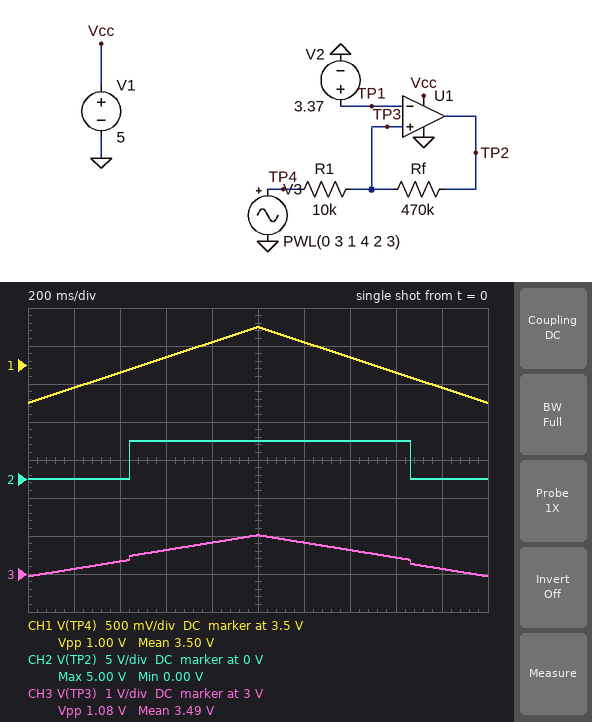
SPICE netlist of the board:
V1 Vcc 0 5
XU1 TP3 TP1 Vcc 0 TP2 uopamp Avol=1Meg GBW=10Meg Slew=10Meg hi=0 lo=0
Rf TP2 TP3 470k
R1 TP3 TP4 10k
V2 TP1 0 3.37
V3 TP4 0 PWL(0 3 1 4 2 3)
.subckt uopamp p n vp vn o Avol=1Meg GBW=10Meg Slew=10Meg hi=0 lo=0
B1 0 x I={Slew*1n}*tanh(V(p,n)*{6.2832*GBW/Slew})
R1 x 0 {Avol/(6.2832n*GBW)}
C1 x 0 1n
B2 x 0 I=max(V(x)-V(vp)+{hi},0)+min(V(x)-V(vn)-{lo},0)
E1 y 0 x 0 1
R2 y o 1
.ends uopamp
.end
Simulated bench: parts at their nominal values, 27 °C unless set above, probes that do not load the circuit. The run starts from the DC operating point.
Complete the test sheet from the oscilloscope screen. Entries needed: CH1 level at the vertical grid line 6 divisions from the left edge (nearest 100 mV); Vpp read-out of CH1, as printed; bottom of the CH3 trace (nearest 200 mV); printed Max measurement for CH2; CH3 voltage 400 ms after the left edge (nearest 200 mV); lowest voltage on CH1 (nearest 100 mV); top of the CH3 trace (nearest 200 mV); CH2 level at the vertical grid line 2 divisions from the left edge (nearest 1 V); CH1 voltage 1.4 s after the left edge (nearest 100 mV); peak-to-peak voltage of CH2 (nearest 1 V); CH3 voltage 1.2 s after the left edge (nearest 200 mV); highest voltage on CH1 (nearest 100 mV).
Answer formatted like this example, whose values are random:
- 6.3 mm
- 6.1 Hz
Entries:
- 3.8 V
- 1.00 V
- 3.0 V
- 5.00 V
- 3.4 V
- 3.0 V
- 4.0 V
- 0 V
- 3.6 V
- 5 V
- 3.8 V
- 4.0 V
